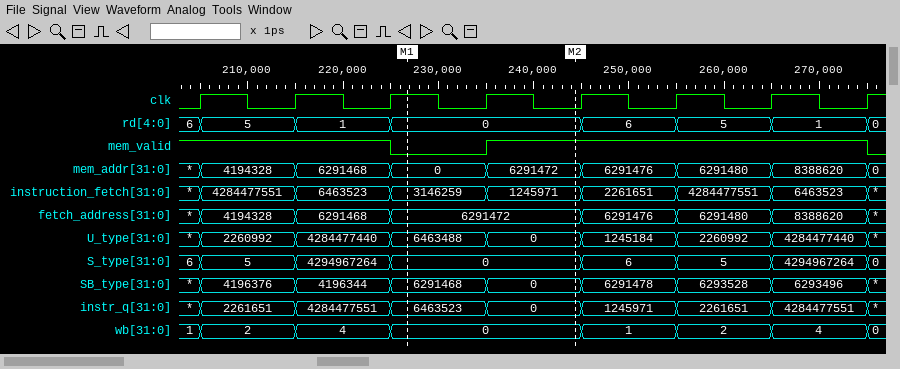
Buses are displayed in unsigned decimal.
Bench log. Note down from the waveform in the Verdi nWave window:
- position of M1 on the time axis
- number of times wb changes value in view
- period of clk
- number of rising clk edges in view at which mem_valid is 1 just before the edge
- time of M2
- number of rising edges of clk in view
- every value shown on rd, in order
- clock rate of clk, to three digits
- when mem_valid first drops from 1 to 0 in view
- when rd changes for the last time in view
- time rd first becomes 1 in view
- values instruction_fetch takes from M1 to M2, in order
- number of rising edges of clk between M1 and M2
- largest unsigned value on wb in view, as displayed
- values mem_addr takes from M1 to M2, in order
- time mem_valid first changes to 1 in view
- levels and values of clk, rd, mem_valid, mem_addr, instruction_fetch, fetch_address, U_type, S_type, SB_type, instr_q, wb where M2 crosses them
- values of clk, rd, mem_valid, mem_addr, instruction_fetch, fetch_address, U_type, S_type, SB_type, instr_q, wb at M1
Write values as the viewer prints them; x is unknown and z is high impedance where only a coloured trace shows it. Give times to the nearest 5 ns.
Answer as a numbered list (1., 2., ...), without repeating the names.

1. 225 ns
2. 7
3. 10 ns
4. 7
5. 245 ns
6. 8
7. 6, 5, 1, 0, 6, 5, 1, 0
8. 100 MHz
9. 225 ns
10. 275 ns
11. 215 ns
12. 3146259, 1245971
13. 1
14. 4
15. 0, 6291472
16. 235 ns
17. clk=0, rd=0, mem_valid=1, mem_addr=6291472, instruction_fetch=1245971, fetch_address=6291472, U_type=0, S_type=0, SB_type=0, instr_q=0, wb=0
18. clk=1, rd=0, mem_valid=0, mem_addr=0, instruction_fetch=3146259, fetch_address=6291472, U_type=6463488, S_type=0, SB_type=6291468, instr_q=6463523, wb=0
